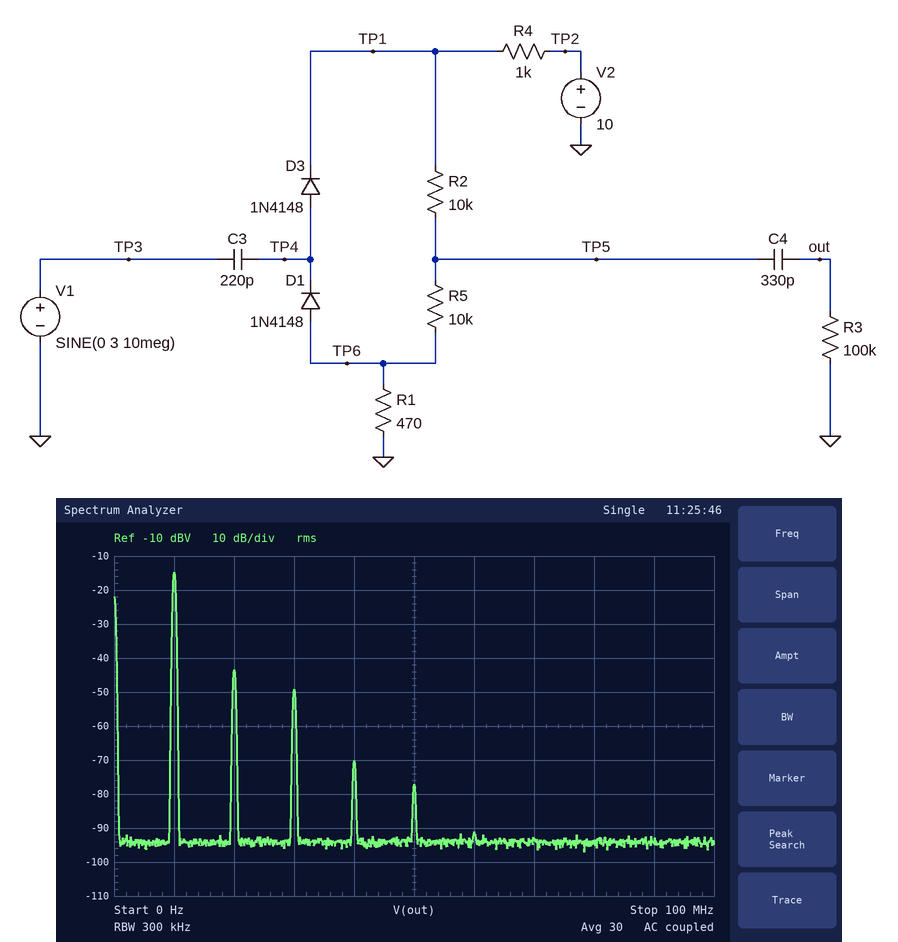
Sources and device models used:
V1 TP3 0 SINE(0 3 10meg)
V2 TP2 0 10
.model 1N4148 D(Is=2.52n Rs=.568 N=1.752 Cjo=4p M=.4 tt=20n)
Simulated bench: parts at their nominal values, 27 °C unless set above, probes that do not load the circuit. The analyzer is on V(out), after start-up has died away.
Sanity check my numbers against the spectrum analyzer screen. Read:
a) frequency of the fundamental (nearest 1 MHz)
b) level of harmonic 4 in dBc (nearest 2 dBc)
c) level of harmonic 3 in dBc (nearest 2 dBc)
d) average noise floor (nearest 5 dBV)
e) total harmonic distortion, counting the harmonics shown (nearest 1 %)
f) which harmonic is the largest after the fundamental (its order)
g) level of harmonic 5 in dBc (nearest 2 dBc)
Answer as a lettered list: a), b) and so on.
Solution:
a) 10 MHz
b) -56 dBc
c) -34 dBc
d) -95 dBV
e) 4 %
f) 2
g) -62 dBc
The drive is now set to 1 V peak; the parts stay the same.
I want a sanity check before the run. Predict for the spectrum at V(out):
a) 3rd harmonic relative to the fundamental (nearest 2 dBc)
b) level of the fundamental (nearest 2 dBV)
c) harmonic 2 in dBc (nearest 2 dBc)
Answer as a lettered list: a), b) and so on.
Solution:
a) -54 dBc
b) -24 dBV
c) -38 dBc
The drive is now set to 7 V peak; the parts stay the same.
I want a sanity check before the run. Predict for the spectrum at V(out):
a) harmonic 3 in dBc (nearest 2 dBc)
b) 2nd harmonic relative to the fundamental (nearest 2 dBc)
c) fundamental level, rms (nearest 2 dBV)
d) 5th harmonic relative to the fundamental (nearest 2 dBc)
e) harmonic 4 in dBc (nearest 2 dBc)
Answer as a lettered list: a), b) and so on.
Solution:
a) -6 dBc
b) -14 dBc
c) -4 dBV
d) -20 dBc
e) -18 dBc
